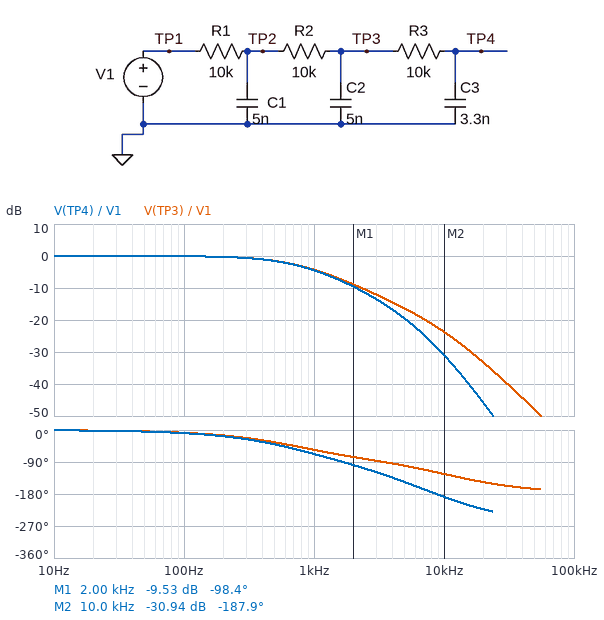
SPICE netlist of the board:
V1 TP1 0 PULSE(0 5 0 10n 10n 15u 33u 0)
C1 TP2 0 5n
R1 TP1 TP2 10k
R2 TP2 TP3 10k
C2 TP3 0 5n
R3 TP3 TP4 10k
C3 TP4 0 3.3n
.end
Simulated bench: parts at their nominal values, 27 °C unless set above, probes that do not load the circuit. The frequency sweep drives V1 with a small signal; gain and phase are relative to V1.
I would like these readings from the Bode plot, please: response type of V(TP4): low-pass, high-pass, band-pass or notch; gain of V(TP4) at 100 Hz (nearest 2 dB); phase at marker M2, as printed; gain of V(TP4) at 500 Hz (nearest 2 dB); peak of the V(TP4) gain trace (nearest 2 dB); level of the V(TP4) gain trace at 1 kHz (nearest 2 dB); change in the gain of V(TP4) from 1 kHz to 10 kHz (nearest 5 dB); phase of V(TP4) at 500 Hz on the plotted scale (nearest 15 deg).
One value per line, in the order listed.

low-pass
0 dB
-187.9 deg
-2 dB
0 dB
-4 dB
-25 dB
-45 deg
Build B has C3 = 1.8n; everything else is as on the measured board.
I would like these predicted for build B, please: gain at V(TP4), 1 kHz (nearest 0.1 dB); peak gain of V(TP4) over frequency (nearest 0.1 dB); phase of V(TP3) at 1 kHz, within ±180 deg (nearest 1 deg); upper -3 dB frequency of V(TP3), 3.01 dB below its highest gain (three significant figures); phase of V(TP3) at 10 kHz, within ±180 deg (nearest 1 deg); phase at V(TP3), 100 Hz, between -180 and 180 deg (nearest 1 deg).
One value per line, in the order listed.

-3.4 dB
0 dB
-53 deg
928 Hz
-127 deg
-7 deg
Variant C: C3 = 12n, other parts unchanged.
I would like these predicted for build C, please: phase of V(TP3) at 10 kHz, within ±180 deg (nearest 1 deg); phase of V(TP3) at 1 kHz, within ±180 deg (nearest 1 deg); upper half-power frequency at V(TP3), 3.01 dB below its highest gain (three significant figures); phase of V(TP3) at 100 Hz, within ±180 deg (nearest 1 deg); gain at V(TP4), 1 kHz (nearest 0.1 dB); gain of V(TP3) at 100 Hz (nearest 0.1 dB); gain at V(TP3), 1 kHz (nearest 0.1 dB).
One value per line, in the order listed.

-120 deg
-54 deg
375 Hz
-14 deg
-9.9 dB
-0.3 dB
-8.0 dB
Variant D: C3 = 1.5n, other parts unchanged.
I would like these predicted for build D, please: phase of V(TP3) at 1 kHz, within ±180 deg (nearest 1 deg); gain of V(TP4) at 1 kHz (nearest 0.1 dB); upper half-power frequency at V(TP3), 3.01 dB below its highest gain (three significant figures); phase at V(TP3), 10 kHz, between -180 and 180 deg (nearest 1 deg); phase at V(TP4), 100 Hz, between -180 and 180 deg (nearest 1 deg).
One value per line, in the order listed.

-52 deg
-3.2 dB
966 Hz
-129 deg
-7 deg
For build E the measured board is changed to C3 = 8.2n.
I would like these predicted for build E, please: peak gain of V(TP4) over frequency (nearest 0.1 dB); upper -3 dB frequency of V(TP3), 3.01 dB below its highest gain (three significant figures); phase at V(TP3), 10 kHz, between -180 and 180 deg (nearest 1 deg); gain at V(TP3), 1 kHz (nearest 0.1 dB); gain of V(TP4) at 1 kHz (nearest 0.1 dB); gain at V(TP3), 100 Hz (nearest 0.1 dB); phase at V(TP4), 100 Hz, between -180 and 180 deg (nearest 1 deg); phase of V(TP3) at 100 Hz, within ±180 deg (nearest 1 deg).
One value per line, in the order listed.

0 dB
486 Hz
-120 deg
-6.8 dB
-7.8 dB
-0.2 dB
-14 deg
-11 deg
